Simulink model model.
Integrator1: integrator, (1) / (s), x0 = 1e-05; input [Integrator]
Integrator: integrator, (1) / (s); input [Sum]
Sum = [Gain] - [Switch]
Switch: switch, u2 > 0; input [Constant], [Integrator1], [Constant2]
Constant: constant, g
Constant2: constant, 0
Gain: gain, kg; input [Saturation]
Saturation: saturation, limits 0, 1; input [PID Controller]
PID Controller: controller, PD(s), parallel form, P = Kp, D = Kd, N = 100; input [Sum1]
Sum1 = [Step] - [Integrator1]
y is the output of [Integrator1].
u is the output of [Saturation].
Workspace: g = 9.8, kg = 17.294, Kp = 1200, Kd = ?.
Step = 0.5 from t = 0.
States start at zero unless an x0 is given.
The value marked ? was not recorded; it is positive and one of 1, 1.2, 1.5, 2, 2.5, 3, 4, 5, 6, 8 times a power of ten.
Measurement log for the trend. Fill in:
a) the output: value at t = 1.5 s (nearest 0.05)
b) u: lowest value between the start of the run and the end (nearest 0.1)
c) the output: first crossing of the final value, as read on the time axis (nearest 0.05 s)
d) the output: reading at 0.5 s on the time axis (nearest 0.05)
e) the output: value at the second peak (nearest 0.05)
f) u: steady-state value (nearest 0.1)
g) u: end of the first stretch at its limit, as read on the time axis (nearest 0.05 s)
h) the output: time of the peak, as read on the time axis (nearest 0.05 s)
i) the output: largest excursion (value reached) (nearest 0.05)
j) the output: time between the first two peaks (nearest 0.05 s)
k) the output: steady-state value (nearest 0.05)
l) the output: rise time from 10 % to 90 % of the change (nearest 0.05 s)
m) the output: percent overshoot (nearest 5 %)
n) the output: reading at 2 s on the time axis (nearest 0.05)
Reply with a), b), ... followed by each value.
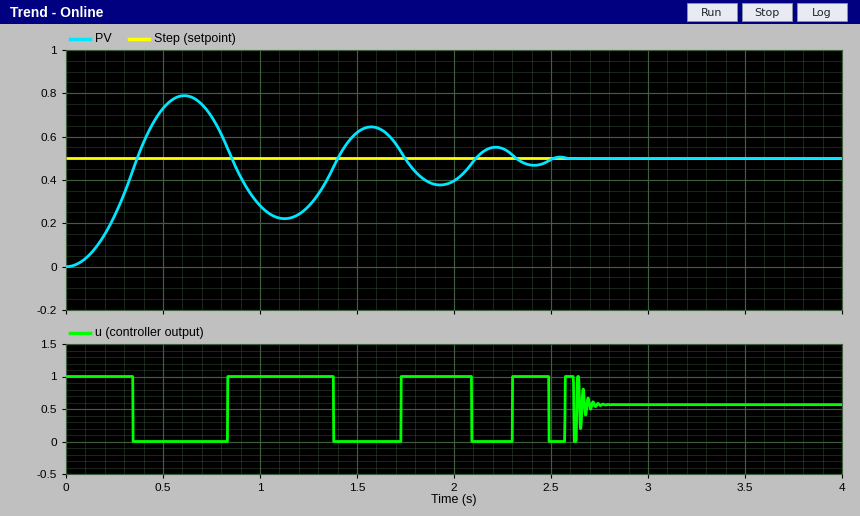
a) 0.60
b) 0.0
c) 0.35 s
d) 0.75
e) 0.65
f) 0.6
g) 0.35 s
h) 0.60 s
i) 0.80
j) 0.95 s
k) 0.50
l) 0.25 s
m) 60 %
n) 0.40
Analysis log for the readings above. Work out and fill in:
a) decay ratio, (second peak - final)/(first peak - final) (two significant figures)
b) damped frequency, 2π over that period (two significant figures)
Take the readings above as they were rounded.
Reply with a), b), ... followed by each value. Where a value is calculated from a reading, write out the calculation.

a) (0.65 - 0.5) / (0.8 - 0.5) = 0.50
b) 2π / 0.95 = 6.6 rad/s
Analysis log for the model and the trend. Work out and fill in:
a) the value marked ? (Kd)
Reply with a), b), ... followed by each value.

a) 25
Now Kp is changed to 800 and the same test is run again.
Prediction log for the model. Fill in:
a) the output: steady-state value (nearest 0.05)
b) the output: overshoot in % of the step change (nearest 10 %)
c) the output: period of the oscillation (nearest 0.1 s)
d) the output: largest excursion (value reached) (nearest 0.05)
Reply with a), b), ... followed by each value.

a) 0.50
b) 50 %
c) 0.8 s
d) 0.75
